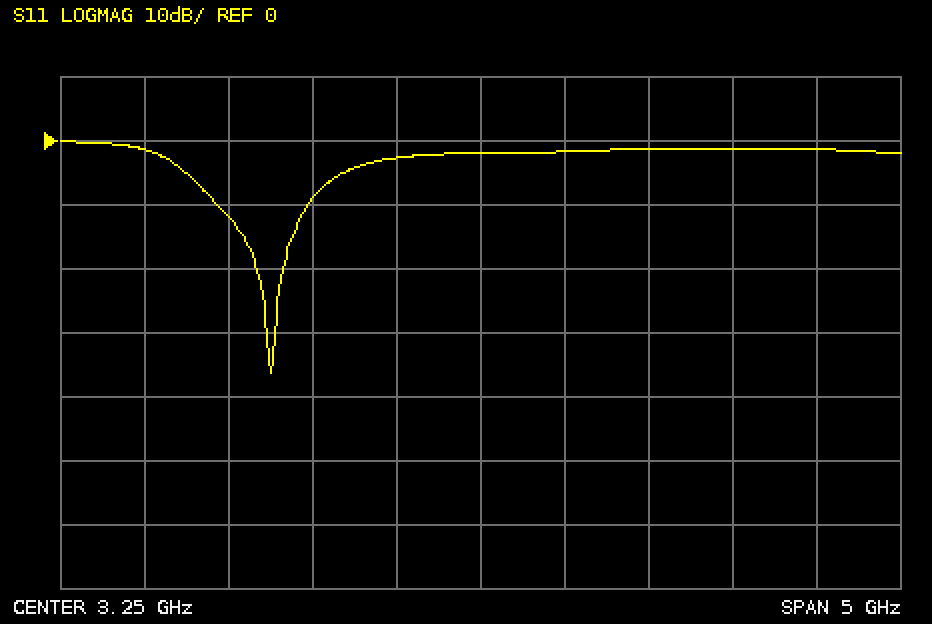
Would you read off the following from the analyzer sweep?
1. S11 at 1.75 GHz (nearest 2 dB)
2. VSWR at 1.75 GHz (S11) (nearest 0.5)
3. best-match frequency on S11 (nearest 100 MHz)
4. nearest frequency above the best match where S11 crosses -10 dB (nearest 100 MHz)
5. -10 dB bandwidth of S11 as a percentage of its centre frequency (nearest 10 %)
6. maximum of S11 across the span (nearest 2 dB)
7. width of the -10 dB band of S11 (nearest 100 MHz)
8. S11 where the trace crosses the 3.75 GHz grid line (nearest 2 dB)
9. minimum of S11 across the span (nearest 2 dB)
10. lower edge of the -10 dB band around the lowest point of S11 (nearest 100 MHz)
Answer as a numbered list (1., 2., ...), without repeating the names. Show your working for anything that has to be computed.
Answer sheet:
1. -12 dB
2. |Γ| = 10^(-12/20) = 0.2512; VSWR = (1 + 0.2512)/(1 − 0.2512) ≈ 1.67, so 1.5 to the nearest 0.5
3. 2.0 GHz
4. 2.2 GHz
5. 500 MHz / 1.95 GHz ≈ 25.6 %, so 30 % to the nearest 10 %
6. 0 dB
7. 2.2 GHz − 1.7 GHz = 500 MHz
8. -2 dB
9. -36 dB
10. 1.7 GHz
